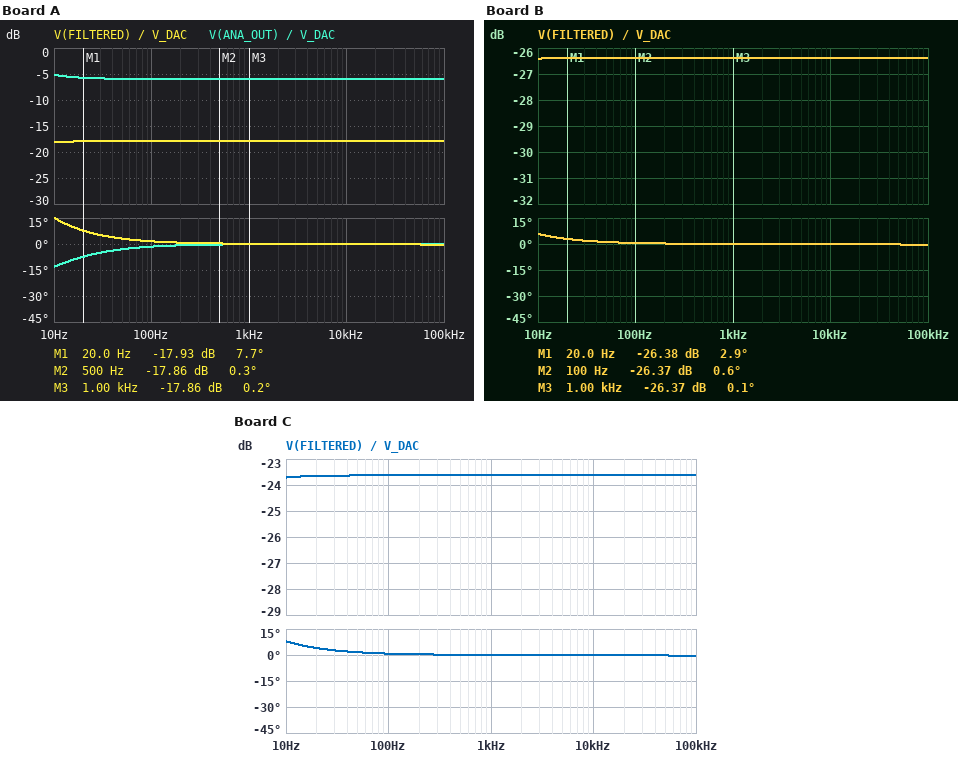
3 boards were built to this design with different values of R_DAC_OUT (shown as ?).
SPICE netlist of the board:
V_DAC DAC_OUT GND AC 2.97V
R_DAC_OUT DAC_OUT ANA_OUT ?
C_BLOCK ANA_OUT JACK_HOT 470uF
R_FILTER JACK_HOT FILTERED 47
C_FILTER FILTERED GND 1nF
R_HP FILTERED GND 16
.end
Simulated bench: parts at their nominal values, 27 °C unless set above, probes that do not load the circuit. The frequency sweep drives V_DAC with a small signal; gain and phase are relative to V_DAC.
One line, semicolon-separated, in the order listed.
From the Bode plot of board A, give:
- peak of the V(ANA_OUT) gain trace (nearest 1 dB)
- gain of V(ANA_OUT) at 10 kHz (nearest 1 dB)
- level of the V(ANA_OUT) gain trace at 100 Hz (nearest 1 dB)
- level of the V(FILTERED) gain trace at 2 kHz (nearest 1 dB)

-5 dB; -6 dB; -6 dB; -18 dB
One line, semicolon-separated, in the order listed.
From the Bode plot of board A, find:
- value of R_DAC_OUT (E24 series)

62 Ω
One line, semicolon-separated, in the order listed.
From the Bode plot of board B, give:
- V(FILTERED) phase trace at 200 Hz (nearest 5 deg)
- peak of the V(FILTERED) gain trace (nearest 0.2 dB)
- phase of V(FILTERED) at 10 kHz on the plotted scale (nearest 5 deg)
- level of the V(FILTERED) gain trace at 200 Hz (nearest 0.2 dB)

0 deg; -26.4 dB; 0 deg; -26.4 dB
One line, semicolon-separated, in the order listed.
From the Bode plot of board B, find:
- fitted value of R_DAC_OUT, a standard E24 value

270 Ω
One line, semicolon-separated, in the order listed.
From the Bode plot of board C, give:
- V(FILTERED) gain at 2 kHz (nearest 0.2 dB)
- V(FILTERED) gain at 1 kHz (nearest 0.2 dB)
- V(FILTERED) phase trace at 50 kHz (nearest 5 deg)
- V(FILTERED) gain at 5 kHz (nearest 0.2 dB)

-23.6 dB; -23.6 dB; 0 deg; -23.6 dB
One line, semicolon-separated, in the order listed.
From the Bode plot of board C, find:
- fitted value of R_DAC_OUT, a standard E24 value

180 Ω
